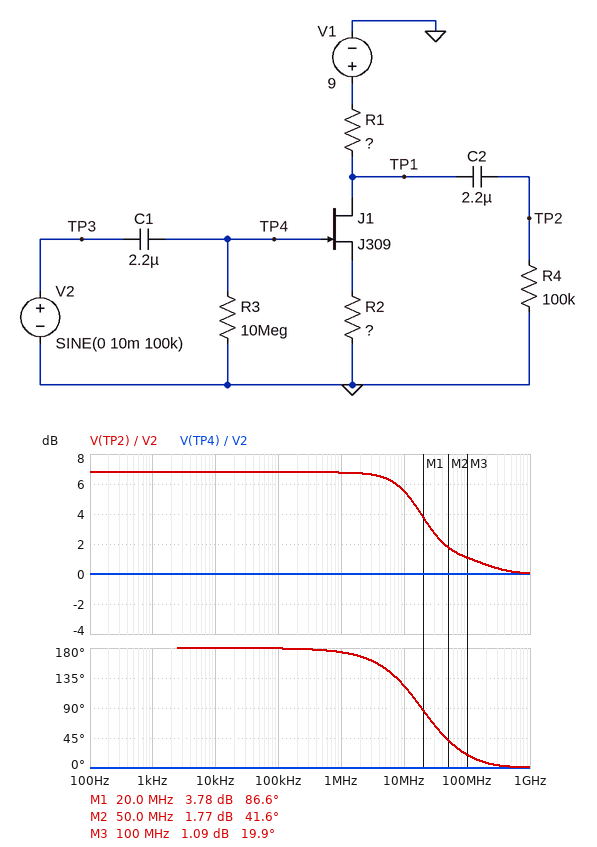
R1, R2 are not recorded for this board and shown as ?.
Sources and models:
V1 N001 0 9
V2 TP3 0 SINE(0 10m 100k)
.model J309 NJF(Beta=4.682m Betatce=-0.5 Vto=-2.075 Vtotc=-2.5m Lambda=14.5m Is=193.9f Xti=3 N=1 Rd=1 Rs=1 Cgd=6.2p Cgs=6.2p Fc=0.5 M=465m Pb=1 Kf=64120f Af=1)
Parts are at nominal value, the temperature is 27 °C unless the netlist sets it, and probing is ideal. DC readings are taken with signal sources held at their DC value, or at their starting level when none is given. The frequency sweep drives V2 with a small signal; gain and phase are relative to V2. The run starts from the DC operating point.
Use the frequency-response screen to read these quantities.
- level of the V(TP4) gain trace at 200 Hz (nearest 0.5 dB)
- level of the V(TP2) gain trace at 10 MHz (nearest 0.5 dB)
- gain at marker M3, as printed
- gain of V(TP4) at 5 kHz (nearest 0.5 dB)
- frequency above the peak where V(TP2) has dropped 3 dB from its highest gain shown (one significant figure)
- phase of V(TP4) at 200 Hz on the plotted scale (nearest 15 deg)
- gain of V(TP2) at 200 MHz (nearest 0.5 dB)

0 dB
5.5 dB
1.09 dB
0 dB
20 MHz
0 deg
0.5 dB
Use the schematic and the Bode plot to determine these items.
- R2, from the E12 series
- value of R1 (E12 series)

1.8 kΩ
4.7 kΩ
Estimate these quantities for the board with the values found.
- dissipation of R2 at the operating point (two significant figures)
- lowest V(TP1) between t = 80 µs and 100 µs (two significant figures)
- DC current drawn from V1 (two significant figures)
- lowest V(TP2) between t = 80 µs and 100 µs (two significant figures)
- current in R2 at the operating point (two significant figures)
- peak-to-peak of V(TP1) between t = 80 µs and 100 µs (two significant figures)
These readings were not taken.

1.5 mW
4.7 V
910 µA
-22 mV
910 µA
44 mV
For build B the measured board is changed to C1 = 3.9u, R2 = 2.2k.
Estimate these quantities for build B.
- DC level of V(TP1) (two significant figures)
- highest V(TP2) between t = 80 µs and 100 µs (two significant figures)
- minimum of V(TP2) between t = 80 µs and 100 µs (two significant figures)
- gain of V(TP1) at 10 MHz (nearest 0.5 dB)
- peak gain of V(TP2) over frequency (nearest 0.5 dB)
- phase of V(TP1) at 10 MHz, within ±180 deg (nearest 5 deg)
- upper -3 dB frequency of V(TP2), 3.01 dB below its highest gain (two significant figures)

5.4 V
18 mV
-18 mV
4.0 dB
5.0 dB
120 deg
30 MHz
